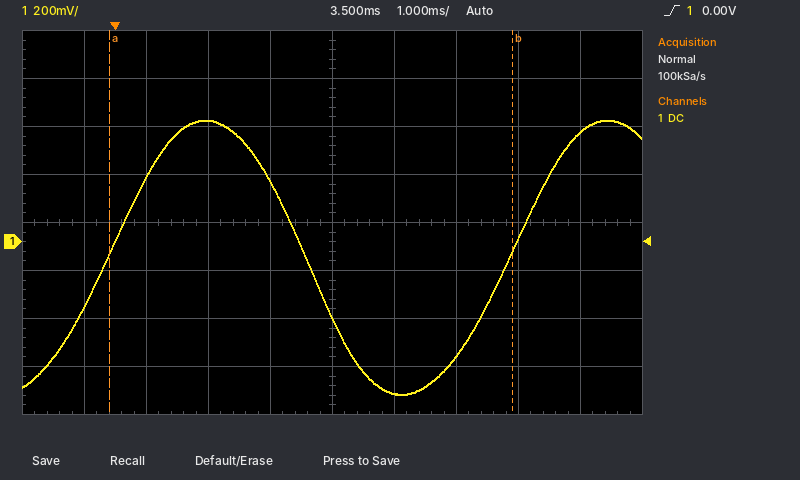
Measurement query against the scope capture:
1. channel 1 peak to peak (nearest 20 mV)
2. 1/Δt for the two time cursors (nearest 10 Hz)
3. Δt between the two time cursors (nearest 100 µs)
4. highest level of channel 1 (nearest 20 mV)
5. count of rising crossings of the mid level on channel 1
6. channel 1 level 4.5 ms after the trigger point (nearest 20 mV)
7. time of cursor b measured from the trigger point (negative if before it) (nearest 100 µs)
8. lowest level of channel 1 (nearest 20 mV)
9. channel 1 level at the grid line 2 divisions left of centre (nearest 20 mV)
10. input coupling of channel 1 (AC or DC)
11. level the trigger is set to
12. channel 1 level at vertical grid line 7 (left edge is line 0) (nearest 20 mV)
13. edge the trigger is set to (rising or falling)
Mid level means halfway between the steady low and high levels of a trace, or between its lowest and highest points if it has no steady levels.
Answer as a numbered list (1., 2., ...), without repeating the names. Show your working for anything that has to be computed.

1. 500 mV − (-640 mV) = 1.14 V
2. 1 / 6.5 ms ≈ 150 Hz
3. 6.5 ms
4. 500 mV
5. 2
6. -640 mV
7. +6.4 ms
8. -640 mV
9. 500 mV
10. DC
11. 0.00 V
12. -480 mV
13. rising
